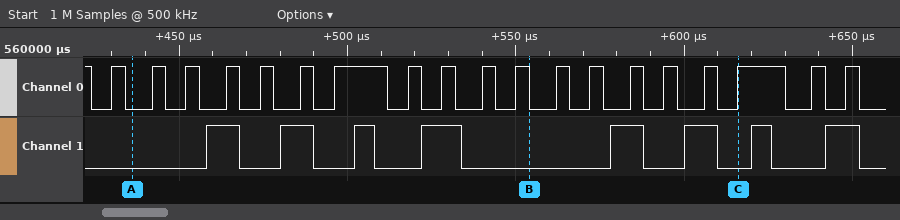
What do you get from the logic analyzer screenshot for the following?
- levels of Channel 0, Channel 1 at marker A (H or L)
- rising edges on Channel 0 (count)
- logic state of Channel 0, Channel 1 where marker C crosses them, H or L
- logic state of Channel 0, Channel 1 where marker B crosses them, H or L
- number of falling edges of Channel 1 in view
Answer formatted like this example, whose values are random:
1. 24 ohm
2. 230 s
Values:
1. Channel 0=L, Channel 1=L
2. 19
3. Channel 0=H, Channel 1=L
4. Channel 0=L, Channel 1=L
5. 8
